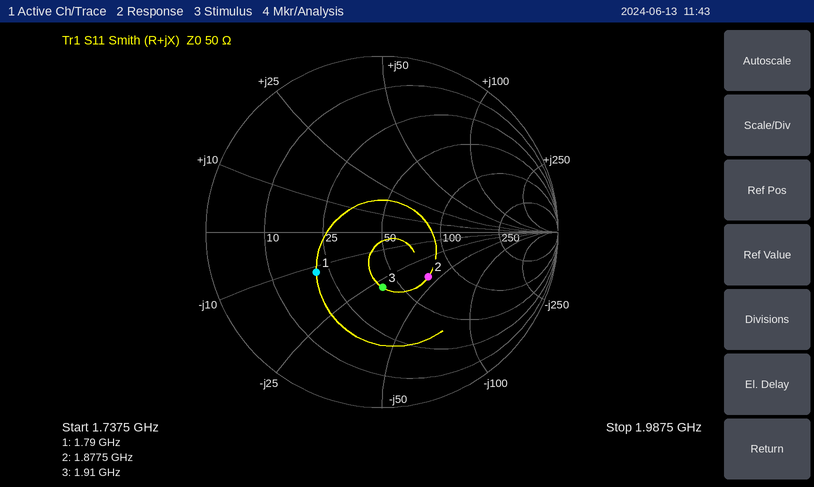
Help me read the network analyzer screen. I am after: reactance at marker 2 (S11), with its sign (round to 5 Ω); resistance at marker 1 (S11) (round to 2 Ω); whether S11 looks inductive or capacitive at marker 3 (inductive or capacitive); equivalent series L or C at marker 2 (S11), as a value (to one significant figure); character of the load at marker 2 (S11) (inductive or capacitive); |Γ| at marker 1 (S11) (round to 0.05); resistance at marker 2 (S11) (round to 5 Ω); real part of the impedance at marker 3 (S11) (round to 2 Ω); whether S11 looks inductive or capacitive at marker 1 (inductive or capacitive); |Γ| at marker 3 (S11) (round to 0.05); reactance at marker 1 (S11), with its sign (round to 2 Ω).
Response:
-40 Ω
20 Ω
capacitive
2 pF
capacitive
0.45
70 Ω
42 Ω
capacitive
0.30
-12 Ω
